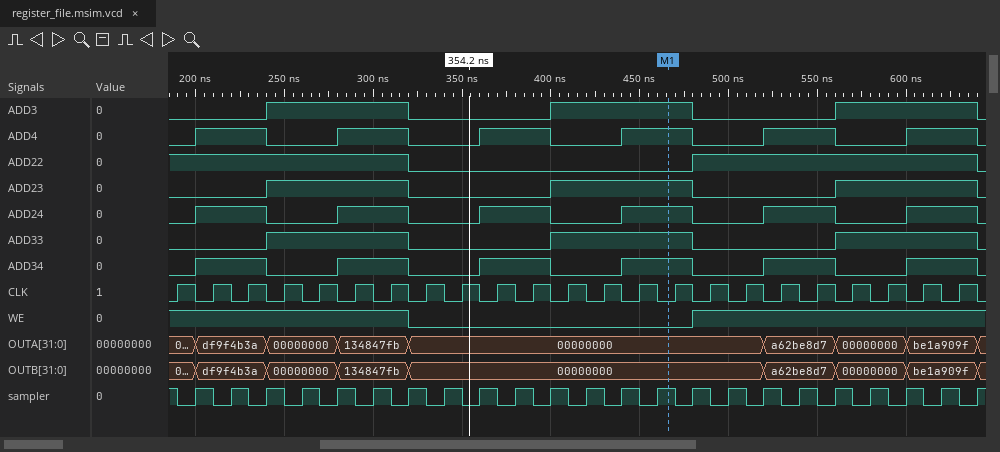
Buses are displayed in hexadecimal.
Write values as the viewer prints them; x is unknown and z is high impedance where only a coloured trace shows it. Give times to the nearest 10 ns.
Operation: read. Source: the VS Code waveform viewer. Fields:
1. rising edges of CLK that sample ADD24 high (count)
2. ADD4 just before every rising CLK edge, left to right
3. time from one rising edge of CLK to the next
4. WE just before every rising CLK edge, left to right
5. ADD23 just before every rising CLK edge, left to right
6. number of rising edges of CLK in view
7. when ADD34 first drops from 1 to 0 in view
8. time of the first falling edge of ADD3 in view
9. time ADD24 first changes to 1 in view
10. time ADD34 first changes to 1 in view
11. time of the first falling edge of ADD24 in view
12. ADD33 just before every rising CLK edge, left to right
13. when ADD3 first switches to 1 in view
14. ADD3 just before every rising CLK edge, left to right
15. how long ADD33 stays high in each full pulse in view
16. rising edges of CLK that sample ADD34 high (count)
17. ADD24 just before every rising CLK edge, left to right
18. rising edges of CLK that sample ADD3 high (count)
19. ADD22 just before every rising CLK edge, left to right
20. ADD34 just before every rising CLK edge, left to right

12
0 1 1 0 0 1 1 0 0 1 1 0 0 1 1 0 0 1 1 0 0 1 1
20 ns
1 1 1 1 1 1 1 0 0 0 0 0 0 0 0 1 1 1 1 1 1 1 1
0 0 0 1 1 1 1 0 0 0 0 1 1 1 1 0 0 0 0 1 1 1 1
23
240 ns
320 ns
200 ns
200 ns
240 ns
0 0 0 1 1 1 1 0 0 0 0 1 1 1 1 0 0 0 0 1 1 1 1
240 ns
0 0 0 1 1 1 1 0 0 0 0 1 1 1 1 0 0 0 0 1 1 1 1
80 ns, 80 ns, 80 ns
12
0 1 1 0 0 1 1 0 0 1 1 0 0 1 1 0 0 1 1 0 0 1 1
12
1 1 1 1 1 1 1 0 0 0 0 0 0 0 0 1 1 1 1 1 1 1 1
0 1 1 0 0 1 1 0 0 1 1 0 0 1 1 0 0 1 1 0 0 1 1
